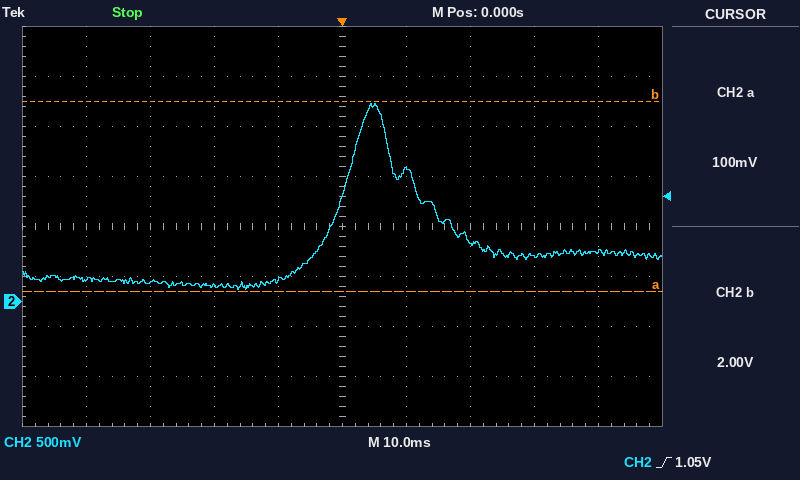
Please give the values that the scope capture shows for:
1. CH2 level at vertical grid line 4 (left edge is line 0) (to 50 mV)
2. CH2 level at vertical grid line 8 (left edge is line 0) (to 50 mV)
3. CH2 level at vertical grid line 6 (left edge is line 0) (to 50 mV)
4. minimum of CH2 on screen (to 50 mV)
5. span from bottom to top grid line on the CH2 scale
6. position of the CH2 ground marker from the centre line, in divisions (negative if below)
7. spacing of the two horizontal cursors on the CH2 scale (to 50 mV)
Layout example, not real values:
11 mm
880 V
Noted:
200 mV
450 mV
1.30 V
100 mV
4 V
-1.5 div
1.90 V
